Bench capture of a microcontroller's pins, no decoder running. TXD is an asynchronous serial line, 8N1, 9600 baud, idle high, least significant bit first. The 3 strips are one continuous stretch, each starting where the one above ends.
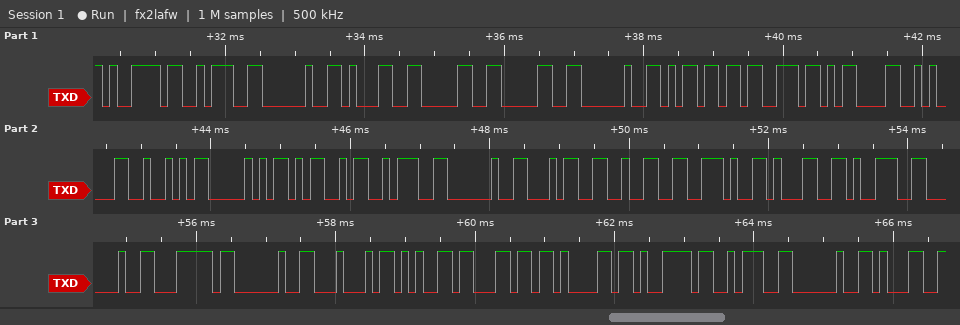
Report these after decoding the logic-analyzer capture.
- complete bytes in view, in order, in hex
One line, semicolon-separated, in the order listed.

79 3A 20 31 30 30 20 6D 73 0D 0A 52 50 4D 3A 20 34 32 2E 31 39 20 7C 20 44 65 6C 61 79 3A 20 31
